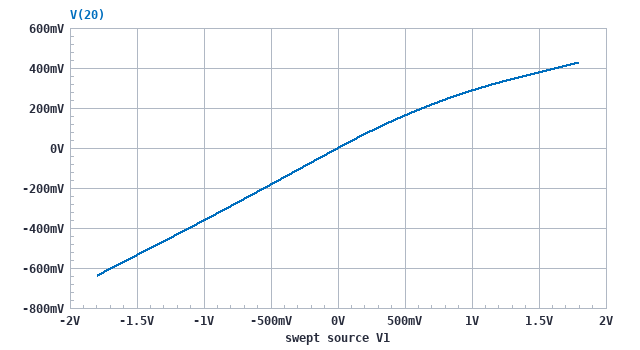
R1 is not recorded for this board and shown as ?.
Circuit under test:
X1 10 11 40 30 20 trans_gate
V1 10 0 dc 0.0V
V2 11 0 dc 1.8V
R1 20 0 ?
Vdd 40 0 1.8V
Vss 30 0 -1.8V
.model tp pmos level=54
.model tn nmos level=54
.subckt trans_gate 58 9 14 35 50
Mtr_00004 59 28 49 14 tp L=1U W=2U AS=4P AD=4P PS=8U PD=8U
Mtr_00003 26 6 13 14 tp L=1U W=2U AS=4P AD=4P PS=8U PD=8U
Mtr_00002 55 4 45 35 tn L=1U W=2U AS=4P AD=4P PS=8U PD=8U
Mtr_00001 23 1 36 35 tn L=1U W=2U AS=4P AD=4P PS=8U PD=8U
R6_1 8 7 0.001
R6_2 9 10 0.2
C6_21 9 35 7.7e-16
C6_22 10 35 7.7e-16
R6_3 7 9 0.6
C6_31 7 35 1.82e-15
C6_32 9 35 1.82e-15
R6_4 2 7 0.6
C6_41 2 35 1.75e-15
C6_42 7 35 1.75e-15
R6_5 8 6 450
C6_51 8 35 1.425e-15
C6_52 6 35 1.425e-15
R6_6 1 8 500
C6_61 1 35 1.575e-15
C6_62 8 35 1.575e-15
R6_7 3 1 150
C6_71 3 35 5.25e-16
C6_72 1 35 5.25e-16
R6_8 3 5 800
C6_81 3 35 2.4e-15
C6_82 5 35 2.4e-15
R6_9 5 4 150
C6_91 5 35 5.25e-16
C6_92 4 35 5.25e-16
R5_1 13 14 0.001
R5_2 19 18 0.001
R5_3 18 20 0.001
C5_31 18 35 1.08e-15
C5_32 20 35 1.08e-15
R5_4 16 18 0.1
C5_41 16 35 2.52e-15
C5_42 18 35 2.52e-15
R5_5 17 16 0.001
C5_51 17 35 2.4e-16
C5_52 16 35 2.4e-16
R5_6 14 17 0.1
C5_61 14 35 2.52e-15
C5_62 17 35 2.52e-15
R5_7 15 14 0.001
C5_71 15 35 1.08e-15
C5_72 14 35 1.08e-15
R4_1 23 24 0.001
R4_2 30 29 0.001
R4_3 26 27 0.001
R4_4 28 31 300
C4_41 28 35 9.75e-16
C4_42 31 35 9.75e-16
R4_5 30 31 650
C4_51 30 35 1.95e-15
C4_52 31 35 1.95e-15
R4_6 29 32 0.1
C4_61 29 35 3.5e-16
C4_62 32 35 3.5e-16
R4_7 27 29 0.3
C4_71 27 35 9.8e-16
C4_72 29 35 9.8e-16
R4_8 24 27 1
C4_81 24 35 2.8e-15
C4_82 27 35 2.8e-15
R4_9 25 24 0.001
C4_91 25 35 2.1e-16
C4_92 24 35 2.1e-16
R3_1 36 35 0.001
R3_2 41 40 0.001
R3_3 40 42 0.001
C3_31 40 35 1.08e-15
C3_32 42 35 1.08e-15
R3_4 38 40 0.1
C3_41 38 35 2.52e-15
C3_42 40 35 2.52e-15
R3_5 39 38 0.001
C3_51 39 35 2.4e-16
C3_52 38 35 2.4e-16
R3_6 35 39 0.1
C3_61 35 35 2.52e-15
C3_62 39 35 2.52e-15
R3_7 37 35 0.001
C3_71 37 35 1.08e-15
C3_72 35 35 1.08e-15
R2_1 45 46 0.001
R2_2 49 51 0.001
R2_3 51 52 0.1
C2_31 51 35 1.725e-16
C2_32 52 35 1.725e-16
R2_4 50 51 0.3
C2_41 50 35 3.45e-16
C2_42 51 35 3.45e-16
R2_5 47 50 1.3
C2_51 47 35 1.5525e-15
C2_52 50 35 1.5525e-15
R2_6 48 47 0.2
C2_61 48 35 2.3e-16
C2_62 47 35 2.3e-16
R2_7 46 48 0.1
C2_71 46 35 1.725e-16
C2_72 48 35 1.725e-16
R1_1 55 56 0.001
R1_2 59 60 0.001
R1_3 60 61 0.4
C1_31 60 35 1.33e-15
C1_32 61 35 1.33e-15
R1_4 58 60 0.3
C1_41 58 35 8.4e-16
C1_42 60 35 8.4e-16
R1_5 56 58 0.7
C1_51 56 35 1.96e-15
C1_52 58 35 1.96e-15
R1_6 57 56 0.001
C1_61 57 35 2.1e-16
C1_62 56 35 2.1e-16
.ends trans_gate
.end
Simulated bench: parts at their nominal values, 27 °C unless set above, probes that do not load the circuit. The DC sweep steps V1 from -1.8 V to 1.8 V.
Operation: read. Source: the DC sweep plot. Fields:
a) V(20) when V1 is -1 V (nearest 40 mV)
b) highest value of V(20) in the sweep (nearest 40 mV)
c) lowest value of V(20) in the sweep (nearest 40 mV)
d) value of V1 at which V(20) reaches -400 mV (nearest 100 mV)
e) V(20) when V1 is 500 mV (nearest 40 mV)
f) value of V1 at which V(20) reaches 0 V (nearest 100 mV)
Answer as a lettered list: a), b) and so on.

a) -360 mV
b) 440 mV
c) -640 mV
d) -1.1 V
e) 160 mV
f) 0 V
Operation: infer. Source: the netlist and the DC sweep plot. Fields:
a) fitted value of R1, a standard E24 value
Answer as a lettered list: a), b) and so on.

a) 390 Ω
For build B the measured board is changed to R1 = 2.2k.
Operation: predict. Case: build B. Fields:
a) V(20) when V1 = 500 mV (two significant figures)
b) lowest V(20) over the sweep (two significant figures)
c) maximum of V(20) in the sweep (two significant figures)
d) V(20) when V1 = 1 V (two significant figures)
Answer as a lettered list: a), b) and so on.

a) 370 mV
b) -1.4 V
c) 1.1 V
d) 690 mV
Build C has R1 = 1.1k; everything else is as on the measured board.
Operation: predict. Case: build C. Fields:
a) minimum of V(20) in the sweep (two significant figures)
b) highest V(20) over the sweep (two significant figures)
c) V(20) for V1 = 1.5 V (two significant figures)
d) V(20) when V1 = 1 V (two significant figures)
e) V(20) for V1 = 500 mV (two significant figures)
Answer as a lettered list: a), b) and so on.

a) -1.1 V
b) 810 mV
c) 710 mV
d) 530 mV
e) 290 mV
